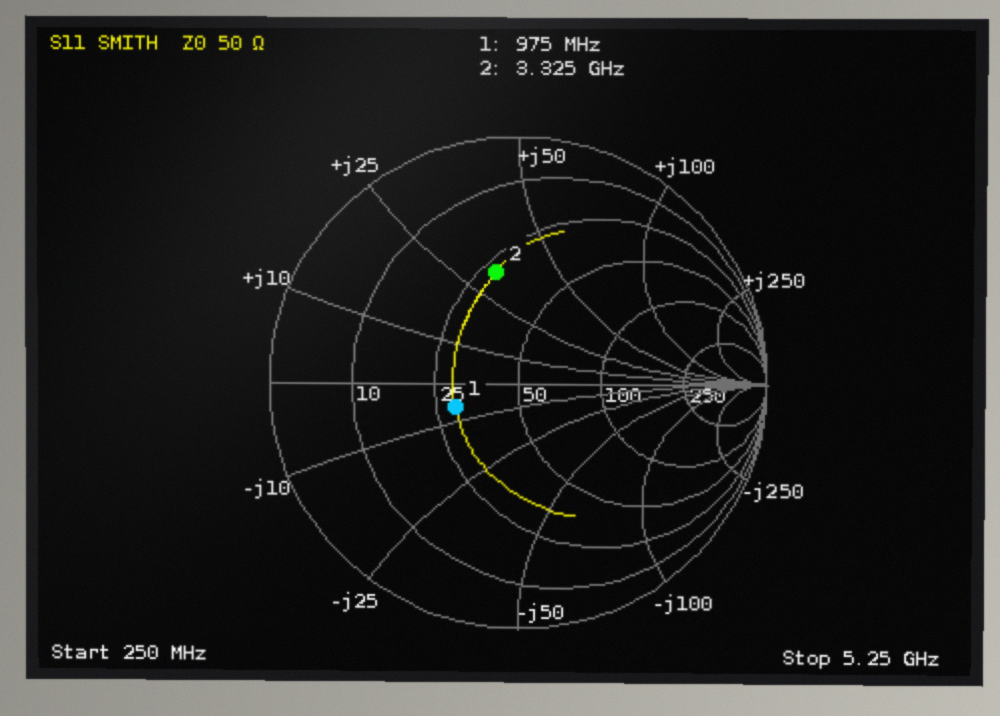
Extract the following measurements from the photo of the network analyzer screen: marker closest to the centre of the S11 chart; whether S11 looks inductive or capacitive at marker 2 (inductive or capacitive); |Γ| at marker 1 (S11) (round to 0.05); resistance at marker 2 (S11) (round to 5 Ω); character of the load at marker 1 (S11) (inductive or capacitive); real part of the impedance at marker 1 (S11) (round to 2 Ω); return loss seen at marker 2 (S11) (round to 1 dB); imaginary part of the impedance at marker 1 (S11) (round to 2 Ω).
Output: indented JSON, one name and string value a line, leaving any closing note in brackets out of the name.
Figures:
{
  "marker closest to the centre of the S11 chart": "marker 1",
  "whether S11 looks inductive or capacitive at marker 2": "inductive",
  "|Γ| at marker 1 (S11)": "0.25",
  "resistance at marker 2 (S11)": "30 Ω",
  "character of the load at marker 1 (S11)": "capacitive",
  "real part of the impedance at marker 1 (S11)": "30 Ω",
  "return loss seen at marker 2 (S11)": "7 dB",
  "imaginary part of the impedance at marker 1 (S11)": "-6 Ω"
}
